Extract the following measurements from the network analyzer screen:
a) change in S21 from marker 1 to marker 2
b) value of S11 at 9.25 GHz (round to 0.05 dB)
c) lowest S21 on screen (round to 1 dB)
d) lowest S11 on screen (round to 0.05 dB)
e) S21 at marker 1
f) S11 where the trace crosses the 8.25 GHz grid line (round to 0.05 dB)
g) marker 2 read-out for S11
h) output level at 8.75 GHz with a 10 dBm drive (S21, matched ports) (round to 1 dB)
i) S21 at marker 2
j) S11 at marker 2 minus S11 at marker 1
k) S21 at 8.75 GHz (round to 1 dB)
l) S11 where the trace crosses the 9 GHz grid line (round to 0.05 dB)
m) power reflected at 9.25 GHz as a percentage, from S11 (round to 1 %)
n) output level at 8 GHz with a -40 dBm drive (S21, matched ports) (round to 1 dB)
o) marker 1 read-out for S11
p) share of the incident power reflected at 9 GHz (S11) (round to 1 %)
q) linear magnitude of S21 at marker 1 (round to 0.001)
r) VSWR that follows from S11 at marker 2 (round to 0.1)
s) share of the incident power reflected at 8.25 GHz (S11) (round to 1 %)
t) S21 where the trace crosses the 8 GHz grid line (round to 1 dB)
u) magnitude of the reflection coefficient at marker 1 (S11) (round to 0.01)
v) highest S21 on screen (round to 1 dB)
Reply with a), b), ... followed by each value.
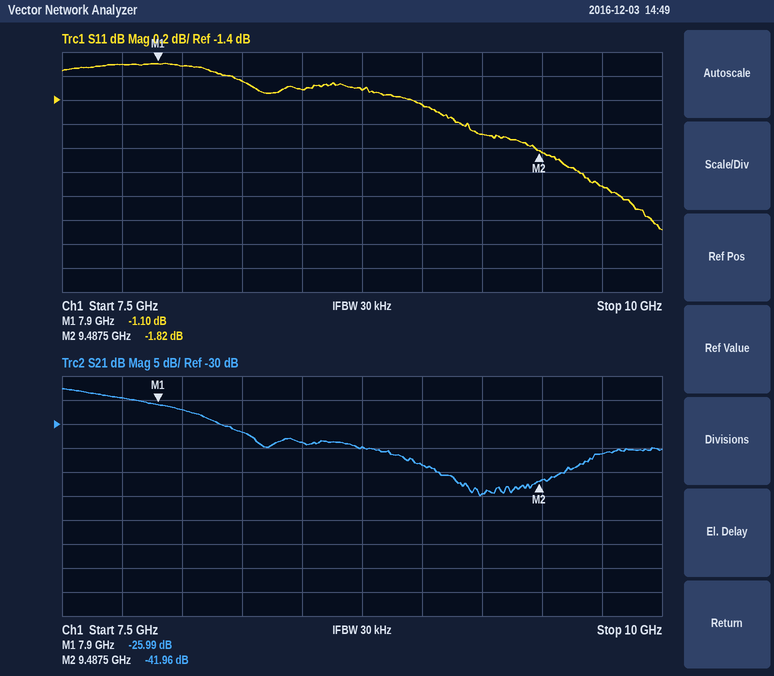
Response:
a) -15.97 dB
b) -1.70 dB
c) -45 dB
d) -2.50 dB
e) -25.99 dB
f) -1.25 dB
g) -1.82 dB
h) -25 dBm
i) -41.96 dB
j) -0.72 dB
k) -35 dB
l) -1.45 dB
m) 68 %
n) -67 dBm
o) -1.10 dB
p) 72 %
q) 0.050
r) 9.6
s) 75 %
t) -27 dB
u) 0.88
v) -23 dB
